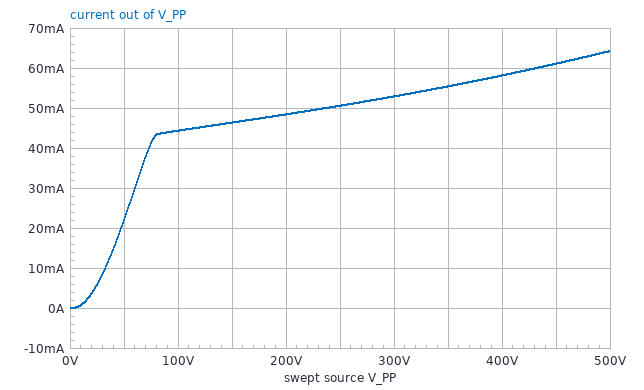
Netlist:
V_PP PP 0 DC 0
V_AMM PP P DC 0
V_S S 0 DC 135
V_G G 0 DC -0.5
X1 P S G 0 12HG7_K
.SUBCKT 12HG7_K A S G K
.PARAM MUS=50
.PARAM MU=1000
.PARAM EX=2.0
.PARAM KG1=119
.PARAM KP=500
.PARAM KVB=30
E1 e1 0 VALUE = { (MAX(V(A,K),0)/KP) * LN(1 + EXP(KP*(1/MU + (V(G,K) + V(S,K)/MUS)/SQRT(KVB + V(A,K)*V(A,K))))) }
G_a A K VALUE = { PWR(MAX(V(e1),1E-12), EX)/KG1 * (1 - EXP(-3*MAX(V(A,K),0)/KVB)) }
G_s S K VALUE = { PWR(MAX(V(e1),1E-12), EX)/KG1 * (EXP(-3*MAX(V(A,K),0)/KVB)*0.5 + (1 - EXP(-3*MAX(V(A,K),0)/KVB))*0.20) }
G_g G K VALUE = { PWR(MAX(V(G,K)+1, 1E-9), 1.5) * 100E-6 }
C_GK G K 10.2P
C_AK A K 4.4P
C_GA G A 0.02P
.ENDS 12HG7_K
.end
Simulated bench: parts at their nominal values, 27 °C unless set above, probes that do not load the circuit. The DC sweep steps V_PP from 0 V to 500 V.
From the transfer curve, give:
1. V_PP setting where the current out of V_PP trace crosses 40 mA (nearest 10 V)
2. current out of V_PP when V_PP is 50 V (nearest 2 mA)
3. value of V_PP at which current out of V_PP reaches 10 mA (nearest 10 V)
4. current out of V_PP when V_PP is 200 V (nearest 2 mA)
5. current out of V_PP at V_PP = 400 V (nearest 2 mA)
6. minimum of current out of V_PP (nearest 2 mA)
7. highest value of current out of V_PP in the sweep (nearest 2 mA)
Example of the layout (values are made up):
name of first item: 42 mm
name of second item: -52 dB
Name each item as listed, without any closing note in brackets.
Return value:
V_PP setting where the current out of V_PP trace crosses 40 mA: 70 V
current out of V_PP when V_PP is 50 V: 22 mA
value of V_PP at which current out of V_PP reaches 10 mA: 30 V
current out of V_PP when V_PP is 200 V: 48 mA
current out of V_PP at V_PP = 400 V: 58 mA
minimum of current out of V_PP: 0 A
highest value of current out of V_PP in the sweep: 64 mA
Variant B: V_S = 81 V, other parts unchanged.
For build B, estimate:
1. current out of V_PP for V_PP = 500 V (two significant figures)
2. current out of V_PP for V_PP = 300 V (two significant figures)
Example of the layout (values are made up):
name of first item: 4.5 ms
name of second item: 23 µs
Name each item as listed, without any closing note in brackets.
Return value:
current out of V_PP for V_PP = 500 V: 27 mA
current out of V_PP for V_PP = 300 V: 18 mA
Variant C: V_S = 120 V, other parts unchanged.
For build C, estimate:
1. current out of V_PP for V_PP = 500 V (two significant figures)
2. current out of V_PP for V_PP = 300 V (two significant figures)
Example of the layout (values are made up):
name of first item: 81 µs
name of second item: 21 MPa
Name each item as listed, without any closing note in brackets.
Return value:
current out of V_PP for V_PP = 500 V: 52 mA
current out of V_PP for V_PP = 300 V: 41 mA
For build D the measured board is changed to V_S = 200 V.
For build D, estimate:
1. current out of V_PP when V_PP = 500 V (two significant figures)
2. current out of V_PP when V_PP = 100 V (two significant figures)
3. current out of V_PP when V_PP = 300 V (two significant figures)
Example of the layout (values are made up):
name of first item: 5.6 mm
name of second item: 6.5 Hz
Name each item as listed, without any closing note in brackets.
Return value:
current out of V_PP when V_PP = 500 V: 140 mA
current out of V_PP when V_PP = 100 V: 82 mA
current out of V_PP when V_PP = 300 V: 120 mA
